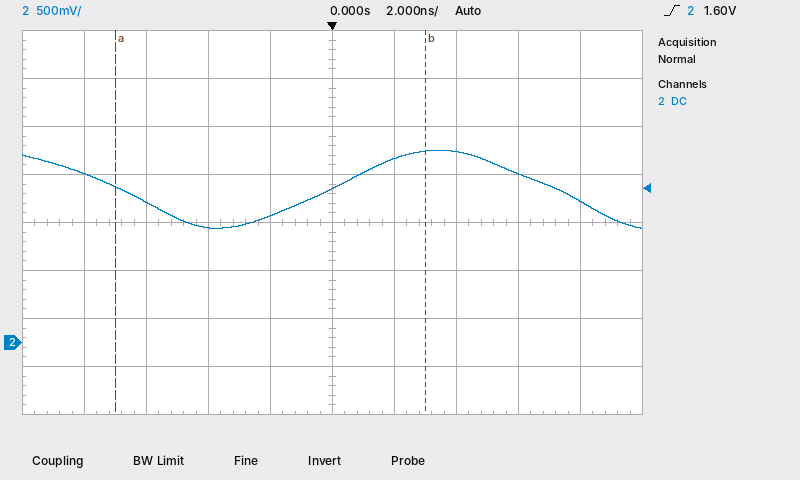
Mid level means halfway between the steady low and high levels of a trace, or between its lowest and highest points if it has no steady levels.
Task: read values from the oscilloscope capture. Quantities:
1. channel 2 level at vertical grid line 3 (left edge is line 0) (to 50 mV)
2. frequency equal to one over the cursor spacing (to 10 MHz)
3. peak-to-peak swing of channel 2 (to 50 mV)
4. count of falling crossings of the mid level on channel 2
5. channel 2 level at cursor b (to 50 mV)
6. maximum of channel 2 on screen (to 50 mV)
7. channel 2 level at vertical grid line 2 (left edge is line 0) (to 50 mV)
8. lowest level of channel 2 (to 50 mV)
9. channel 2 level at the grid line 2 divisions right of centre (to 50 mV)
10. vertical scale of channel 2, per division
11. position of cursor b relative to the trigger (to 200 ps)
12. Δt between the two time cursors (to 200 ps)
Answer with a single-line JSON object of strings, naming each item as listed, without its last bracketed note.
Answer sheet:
{"channel 2 level at vertical grid line 3 (left edge is line 0)": "1.20 V", "frequency equal to one over the cursor spacing": "100 MHz", "peak-to-peak swing of channel 2": "800 mV", "count of falling crossings of the mid level on channel 2": "2", "channel 2 level at cursor b": "2.00 V", "maximum of channel 2 on screen": "2.00 V", "channel 2 level at vertical grid line 2 (left edge is line 0)": "1.45 V", "lowest level of channel 2": "1.20 V", "channel 2 level at the grid line 2 divisions right of centre": "2.00 V", "vertical scale of channel 2, per division": "500 mV", "position of cursor b relative to the trigger": "+3.0 ns", "Δt between the two time cursors": "10.0 ns"}
